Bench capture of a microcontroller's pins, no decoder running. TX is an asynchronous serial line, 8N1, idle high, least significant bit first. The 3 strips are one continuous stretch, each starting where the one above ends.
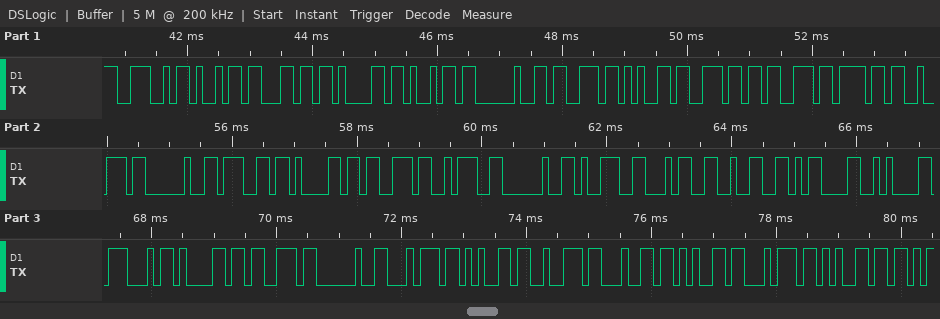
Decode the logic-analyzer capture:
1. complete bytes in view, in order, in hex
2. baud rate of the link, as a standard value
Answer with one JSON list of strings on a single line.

["4E 69 6C 61 69 20 73 65 6E 73 6F 72 20 67 61 73 3A 20 39 34 32 0D 0A 47 61 73 20 74 65 72 64 65 74 65", "9600 baud"]
